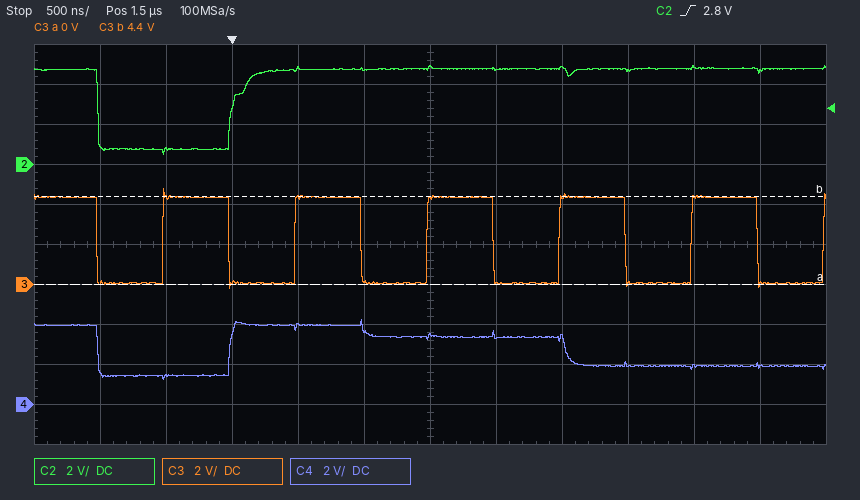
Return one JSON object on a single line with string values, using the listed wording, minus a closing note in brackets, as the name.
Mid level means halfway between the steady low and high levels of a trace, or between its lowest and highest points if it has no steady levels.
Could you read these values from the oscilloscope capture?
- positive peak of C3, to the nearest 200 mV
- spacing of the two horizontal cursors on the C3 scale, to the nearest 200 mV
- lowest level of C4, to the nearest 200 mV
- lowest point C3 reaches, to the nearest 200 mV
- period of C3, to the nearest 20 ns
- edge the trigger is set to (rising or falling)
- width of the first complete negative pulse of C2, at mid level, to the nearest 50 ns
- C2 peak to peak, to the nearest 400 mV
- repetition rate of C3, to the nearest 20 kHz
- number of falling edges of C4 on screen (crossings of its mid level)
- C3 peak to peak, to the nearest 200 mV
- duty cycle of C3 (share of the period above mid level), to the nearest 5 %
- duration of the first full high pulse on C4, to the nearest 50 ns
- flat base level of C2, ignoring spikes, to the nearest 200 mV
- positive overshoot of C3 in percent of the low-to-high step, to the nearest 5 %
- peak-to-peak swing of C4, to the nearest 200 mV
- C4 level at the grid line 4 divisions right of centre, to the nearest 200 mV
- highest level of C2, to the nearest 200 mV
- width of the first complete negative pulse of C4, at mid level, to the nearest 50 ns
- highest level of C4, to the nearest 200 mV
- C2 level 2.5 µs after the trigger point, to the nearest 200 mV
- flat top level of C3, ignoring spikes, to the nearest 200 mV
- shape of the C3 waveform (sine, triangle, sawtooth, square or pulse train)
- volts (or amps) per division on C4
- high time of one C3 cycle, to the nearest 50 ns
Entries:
{"positive peak of C3, to the nearest 200 mV": "4.8 V", "spacing of the two horizontal cursors on the C3 scale, to the nearest 200 mV": "4.4 V", "lowest level of C4, to the nearest 200 mV": "1.2 V", "lowest point C3 reaches, to the nearest 200 mV": "-200 mV", "period of C3, to the nearest 20 ns": "1.00 µs", "edge the trigger is set to": "rising", "width of the first complete negative pulse of C2, at mid level, to the nearest 50 ns": "1.00 µs", "C2 peak to peak, to the nearest 400 mV": "4.4 V", "repetition rate of C3, to the nearest 20 kHz": "1.00 MHz", "number of falling edges of C4 on screen": "2", "C3 peak to peak, to the nearest 200 mV": "5.0 V", "duty cycle of C3 (share of the period above mid level), to the nearest 5 %": "50 %", "duration of the first full high pulse on C4, to the nearest 50 ns": "2.55 µs", "flat base level of C2, ignoring spikes, to the nearest 200 mV": "800 mV", "positive overshoot of C3 in percent of the low-to-high step, to the nearest 5 %": "10 %", "peak-to-peak swing of C4, to the nearest 200 mV": "3.0 V", "C4 level at the grid line 4 divisions right of centre, to the nearest 200 mV": "1.8 V", "highest level of C2, to the nearest 200 mV": "5.0 V", "width of the first complete negative pulse of C4, at mid level, to the nearest 50 ns": "1.00 µs", "highest level of C4, to the nearest 200 mV": "4.2 V", "C2 level 2.5 µs after the trigger point, to the nearest 200 mV": "4.8 V", "flat top level of C3, ignoring spikes, to the nearest 200 mV": "4.4 V", "shape of the C3 waveform": "square", "volts (or amps) per division on C4": "2 V", "high time of one C3 cycle, to the nearest 50 ns": "500 ns"}
